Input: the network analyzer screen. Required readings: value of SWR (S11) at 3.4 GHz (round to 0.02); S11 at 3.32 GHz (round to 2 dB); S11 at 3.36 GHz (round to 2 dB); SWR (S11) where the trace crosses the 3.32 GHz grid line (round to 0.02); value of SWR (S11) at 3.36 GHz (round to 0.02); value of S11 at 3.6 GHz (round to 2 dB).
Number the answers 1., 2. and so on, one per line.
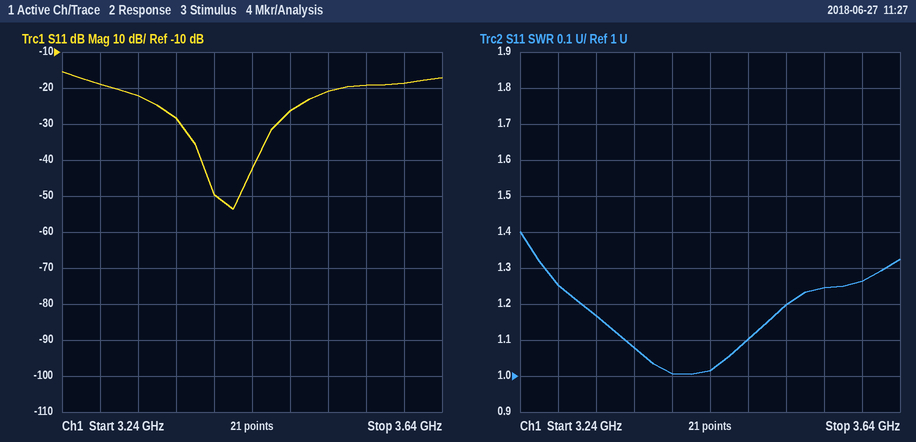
1. 1.00
2. -22 dB
3. -28 dB
4. 1.16
5. 1.08
6. -18 dB
